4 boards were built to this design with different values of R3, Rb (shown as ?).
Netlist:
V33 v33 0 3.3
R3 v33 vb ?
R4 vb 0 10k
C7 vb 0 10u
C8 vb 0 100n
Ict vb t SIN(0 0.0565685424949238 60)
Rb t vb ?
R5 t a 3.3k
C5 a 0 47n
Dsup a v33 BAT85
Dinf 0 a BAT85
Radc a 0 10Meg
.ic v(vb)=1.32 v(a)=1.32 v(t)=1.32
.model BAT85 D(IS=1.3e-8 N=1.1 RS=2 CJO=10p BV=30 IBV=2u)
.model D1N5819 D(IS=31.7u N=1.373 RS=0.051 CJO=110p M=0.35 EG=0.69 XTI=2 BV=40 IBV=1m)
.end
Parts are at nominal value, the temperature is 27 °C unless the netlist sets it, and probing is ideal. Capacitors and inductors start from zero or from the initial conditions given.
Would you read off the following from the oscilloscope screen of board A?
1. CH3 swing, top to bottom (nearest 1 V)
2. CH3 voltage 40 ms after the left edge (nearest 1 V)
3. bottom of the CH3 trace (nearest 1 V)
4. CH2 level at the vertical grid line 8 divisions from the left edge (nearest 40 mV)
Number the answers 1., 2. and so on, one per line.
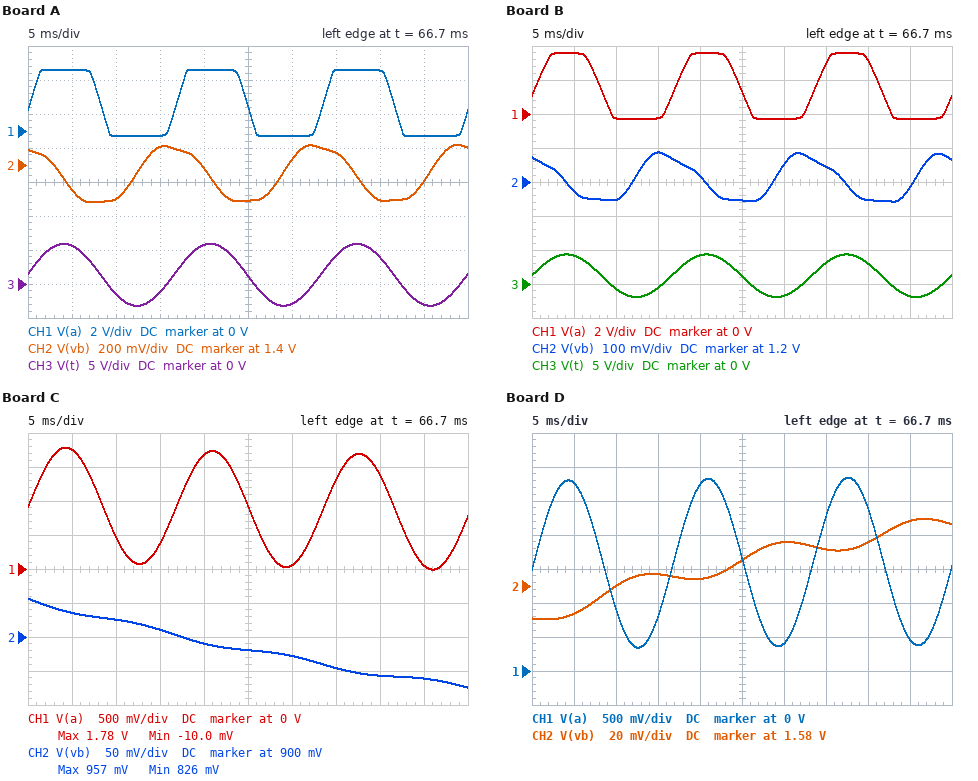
1. 9 V
2. 4 V
3. -3 V
4. 1.20 V
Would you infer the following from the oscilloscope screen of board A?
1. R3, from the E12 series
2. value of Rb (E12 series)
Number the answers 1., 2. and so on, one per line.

1. 27 kΩ
2. 82 Ω
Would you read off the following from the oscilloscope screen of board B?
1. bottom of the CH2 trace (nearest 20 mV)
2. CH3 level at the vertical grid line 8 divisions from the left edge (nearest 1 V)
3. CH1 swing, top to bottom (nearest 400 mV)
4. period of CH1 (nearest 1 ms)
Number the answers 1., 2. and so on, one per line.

1. 1.14 V
2. 3 V
3. 4.0 V
4. 17 ms
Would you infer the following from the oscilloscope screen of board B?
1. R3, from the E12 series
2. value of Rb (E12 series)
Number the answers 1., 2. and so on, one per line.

1. 47 kΩ
2. 56 Ω
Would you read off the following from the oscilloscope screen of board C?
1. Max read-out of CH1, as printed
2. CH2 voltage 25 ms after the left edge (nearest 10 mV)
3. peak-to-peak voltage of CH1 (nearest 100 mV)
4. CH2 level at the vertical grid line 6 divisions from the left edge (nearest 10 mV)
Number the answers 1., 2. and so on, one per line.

1. 1.78 V
2. 880 mV
3. 1.8 V
4. 870 mV
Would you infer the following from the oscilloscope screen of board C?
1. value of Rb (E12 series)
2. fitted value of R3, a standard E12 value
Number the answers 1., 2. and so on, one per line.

1. 15 Ω
2. 39 kΩ
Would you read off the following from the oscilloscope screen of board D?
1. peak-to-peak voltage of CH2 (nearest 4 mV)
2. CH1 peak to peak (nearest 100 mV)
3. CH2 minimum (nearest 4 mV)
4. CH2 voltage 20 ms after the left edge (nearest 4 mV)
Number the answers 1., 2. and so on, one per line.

1. 60 mV
2. 2.5 V
3. 1.560 V
4. 1.584 V
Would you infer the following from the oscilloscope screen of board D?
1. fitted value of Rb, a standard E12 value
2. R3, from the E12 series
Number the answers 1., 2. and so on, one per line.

1. 22 Ω
2. 10 kΩ
